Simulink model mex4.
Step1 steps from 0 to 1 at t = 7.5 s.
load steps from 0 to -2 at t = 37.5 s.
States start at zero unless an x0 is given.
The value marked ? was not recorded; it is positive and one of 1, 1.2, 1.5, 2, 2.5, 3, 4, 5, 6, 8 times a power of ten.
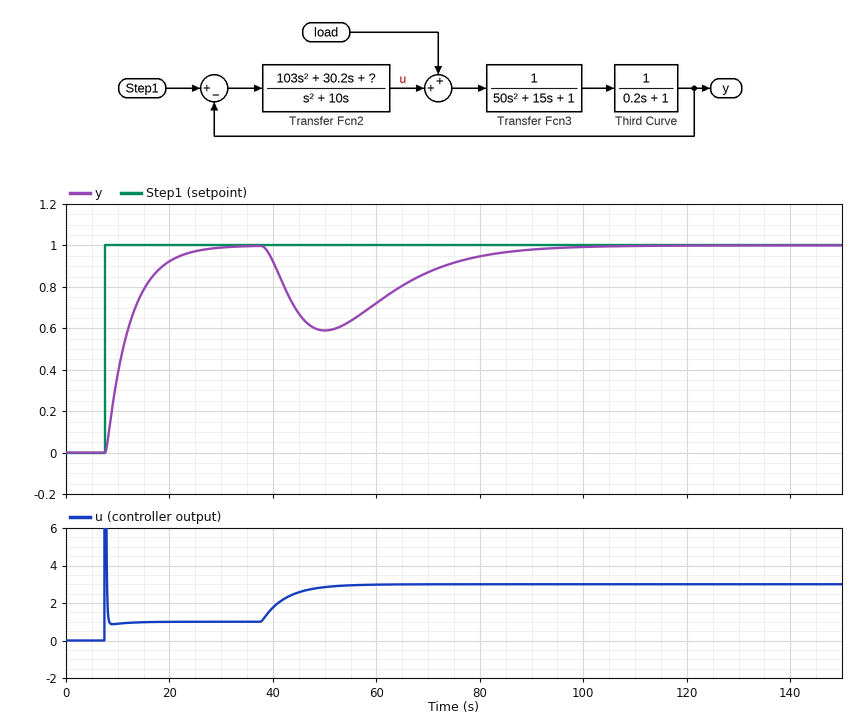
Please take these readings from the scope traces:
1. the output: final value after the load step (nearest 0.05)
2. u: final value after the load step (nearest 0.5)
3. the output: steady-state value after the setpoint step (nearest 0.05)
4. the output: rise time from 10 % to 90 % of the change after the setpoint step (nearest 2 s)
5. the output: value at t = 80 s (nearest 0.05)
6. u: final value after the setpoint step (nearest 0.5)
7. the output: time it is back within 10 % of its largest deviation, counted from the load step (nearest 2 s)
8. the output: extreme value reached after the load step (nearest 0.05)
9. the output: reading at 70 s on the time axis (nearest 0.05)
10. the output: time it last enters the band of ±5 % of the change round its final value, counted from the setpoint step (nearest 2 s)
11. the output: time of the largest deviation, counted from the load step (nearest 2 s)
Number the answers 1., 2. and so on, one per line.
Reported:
1. 1.00
2. 3.0
3. 1.00
4. 10 s
5. 0.95
6. 1.0
7. 46 s
8. 0.60
9. 0.85
10. 14 s
11. 12 s
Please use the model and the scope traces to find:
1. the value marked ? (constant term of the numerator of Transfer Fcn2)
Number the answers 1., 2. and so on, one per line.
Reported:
1. 2
